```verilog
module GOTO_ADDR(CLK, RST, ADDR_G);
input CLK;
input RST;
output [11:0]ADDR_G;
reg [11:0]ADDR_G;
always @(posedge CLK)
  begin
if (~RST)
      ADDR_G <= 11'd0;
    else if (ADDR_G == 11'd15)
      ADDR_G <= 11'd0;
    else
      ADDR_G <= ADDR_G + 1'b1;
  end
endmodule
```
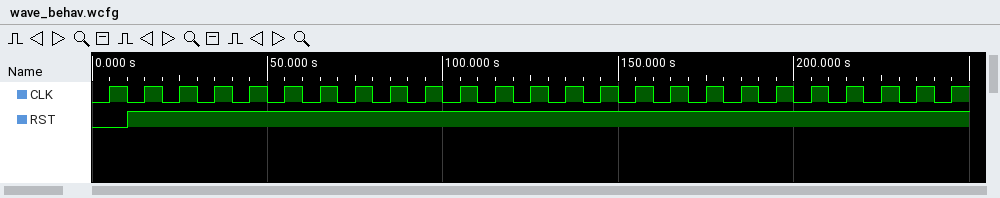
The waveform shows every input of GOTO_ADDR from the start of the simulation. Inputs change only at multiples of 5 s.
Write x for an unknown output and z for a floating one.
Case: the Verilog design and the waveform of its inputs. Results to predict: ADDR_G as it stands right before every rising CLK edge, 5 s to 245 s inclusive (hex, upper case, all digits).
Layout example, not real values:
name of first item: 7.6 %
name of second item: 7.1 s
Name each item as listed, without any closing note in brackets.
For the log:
ADDR_G as it stands right before every rising CLK edge, 5 s to 245 s inclusive: x, 000, 001, 002, 003, 004, 005, 006, 007, 008, 009, 00A, 00B, 00C, 00D, 00E, 00F, 000, 001, 002, 003, 004, 005, 006, 007
